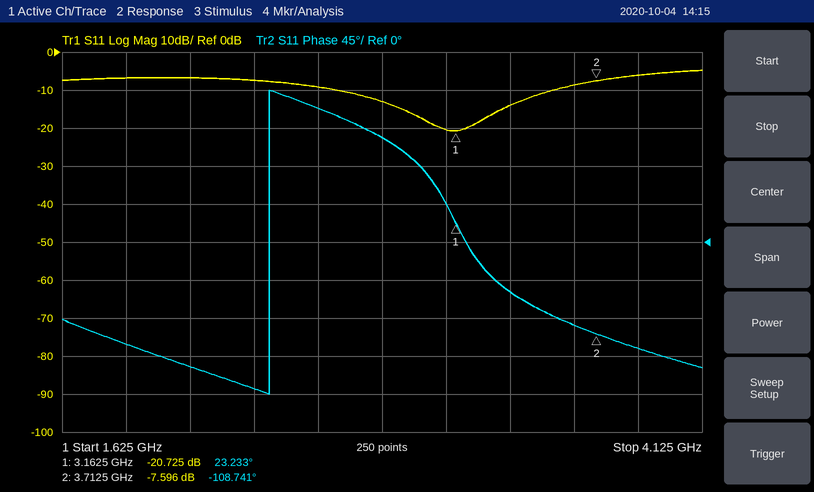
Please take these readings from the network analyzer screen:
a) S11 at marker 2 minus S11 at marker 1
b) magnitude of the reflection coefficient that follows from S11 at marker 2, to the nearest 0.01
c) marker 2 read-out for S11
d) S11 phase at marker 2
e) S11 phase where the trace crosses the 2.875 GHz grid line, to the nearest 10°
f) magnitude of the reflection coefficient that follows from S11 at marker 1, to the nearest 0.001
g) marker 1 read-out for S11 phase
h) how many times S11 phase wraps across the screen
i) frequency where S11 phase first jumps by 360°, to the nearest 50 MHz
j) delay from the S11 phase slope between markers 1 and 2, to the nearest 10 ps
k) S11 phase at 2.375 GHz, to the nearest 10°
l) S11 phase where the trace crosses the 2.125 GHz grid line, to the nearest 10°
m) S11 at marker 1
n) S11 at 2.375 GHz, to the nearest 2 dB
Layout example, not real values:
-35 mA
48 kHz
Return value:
13.129 dB
0.42
-7.596 dB
-108.741°
120°
0.092
23.233°
1
2.45 GHz
670 ps
-170°
-150°
-20.725 dB
-8 dB
